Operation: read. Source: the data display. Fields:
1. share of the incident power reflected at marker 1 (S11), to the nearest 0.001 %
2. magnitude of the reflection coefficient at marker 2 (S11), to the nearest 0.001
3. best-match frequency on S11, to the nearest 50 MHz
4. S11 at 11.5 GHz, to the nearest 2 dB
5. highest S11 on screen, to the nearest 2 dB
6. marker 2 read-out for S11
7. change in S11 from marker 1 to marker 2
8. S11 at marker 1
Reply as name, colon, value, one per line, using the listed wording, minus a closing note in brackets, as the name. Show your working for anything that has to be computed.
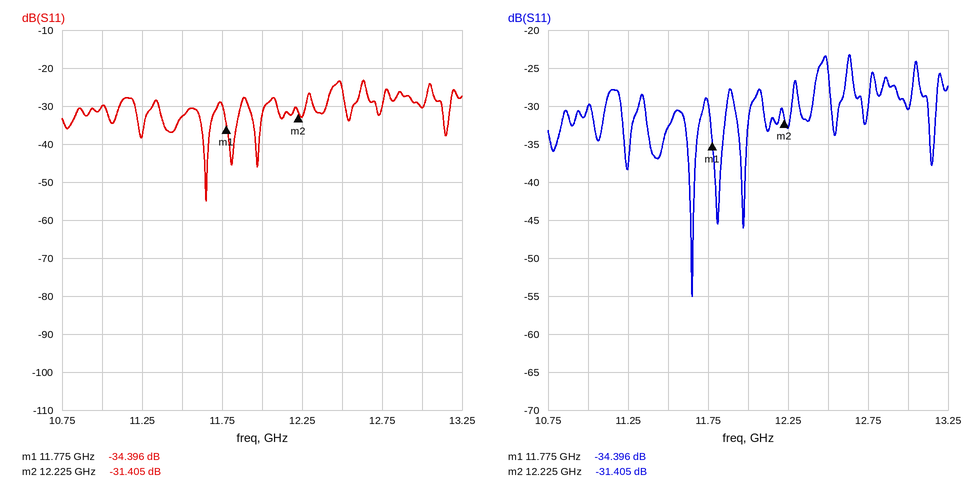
share of the incident power reflected at marker 1 (S11), to the nearest 0.001 %: 10^(-34.396/10) ≈ 0.036 %
magnitude of the reflection coefficient at marker 2 (S11), to the nearest 0.001: 10^(-31.405/20) ≈ 0.027
best-match frequency on S11, to the nearest 50 MHz: 11.65 GHz
S11 at 11.5 GHz, to the nearest 2 dB: -32 dB
highest S11 on screen, to the nearest 2 dB: -24 dB
marker 2 read-out for S11: -31.405 dB
change in S11 from marker 1 to marker 2: -31.405 − (-34.396) = 2.991 dB
S11 at marker 1: -34.396 dB
